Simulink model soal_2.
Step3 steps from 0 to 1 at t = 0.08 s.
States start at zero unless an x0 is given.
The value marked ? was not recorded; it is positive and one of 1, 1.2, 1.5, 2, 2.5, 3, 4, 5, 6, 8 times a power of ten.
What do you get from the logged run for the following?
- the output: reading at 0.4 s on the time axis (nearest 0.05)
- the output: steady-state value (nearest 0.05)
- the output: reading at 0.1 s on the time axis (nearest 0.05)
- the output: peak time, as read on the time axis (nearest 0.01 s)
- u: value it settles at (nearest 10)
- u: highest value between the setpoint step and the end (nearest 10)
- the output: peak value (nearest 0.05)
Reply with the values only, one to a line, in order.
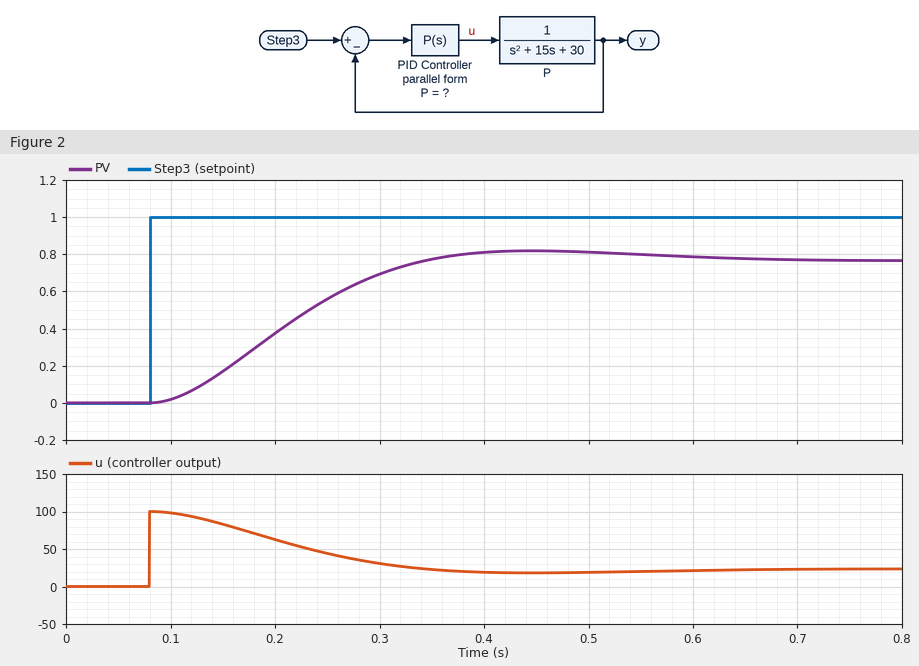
0.80
0.75
0.00
0.45 s
20
100
0.80
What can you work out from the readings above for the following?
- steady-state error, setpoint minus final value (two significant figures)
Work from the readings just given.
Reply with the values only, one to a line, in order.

0.25
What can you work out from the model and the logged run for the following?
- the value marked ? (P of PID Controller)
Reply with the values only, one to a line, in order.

100
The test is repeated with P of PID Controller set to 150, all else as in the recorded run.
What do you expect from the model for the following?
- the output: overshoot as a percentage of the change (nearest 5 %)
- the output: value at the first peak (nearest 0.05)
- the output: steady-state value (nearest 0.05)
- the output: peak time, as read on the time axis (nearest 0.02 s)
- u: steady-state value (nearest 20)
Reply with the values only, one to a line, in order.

10 %
0.95
0.85
0.36 s
20
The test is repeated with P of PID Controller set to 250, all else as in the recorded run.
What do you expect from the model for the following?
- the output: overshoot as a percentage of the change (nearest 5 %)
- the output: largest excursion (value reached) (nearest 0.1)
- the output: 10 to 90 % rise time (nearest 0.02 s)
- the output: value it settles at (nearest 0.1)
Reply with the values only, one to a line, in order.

20 %
1.1
0.10 s
0.9
